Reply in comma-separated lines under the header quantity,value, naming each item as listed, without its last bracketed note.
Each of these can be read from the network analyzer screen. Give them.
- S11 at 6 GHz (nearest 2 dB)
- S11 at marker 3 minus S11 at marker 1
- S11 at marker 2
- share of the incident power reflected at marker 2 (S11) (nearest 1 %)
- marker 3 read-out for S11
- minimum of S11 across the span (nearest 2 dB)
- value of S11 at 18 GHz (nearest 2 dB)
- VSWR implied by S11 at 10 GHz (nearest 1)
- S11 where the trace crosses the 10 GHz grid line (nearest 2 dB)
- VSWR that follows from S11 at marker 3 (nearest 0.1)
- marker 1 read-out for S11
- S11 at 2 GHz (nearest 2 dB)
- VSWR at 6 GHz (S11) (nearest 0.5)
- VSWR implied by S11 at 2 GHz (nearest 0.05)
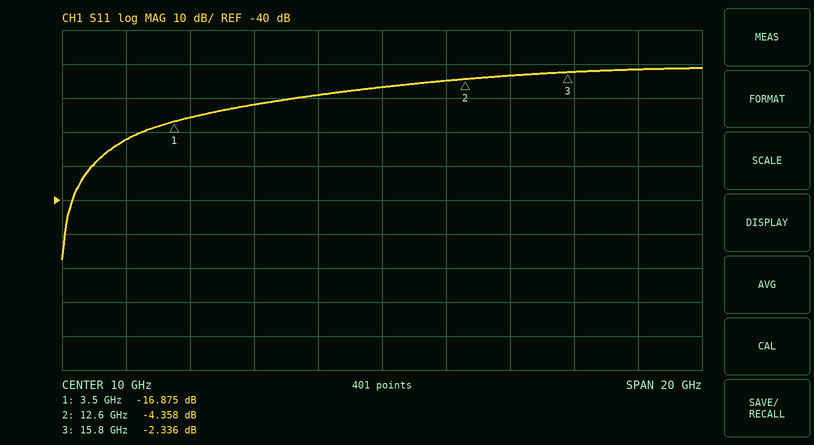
quantity,value
S11 at 6 GHz,-12 dB
S11 at marker 3 minus S11 at marker 1,14.539 dB
S11 at marker 2,-4.358 dB
share of the incident power reflected at marker 2 (S11),37 %
marker 3 read-out for S11,-2.336 dB
minimum of S11 across the span,-58 dB
value of S11 at 18 GHz,-2 dB
VSWR implied by S11 at 10 GHz,3
S11 where the trace crosses the 10 GHz grid line,-6 dB
VSWR that follows from S11 at marker 3,7.5
marker 1 read-out for S11,-16.875 dB
S11 at 2 GHz,-22 dB
VSWR at 6 GHz (S11),1.5
VSWR implied by S11 at 2 GHz,1.15
